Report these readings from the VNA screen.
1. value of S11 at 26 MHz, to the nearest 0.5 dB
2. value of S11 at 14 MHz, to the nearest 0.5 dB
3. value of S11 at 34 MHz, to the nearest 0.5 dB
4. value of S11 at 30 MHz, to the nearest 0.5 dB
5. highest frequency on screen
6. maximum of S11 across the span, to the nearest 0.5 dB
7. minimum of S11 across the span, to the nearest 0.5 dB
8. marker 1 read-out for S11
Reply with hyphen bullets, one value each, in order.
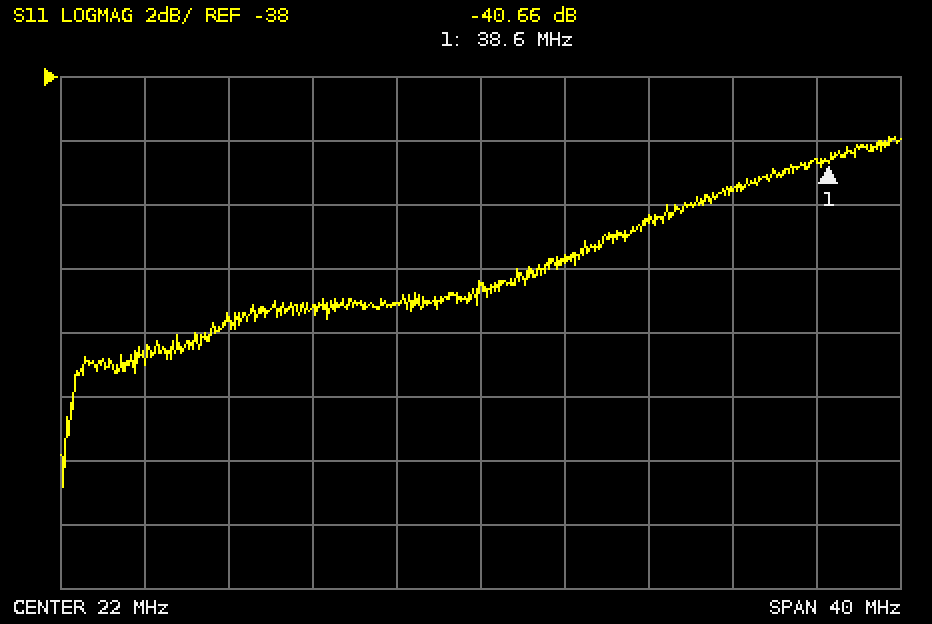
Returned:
- -43.5 dB
- -45.0 dB
- -41.5 dB
- -42.5 dB
- 42 MHz
- -40.0 dB
- -51.0 dB
- -40.66 dB
